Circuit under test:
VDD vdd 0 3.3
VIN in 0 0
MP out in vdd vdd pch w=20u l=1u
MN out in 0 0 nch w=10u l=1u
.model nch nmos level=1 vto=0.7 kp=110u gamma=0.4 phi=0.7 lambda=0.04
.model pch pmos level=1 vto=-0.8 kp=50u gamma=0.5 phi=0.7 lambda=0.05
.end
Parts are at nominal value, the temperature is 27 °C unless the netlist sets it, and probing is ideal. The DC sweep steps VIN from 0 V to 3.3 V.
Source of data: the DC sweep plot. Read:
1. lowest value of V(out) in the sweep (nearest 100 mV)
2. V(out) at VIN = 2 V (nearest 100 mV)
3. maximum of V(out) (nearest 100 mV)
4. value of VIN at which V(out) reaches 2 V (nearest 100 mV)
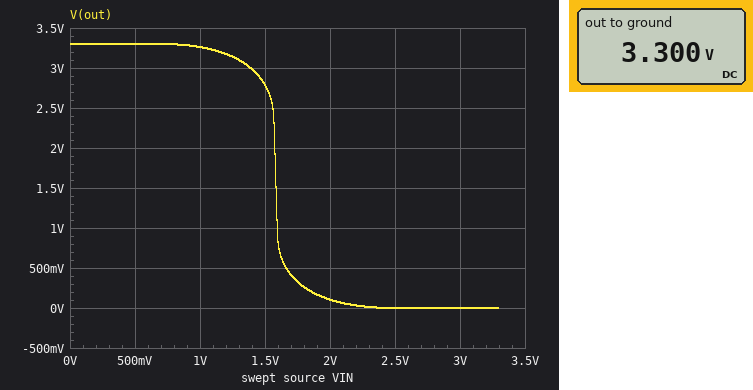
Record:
0 V
100 mV
3.3 V
1.6 V
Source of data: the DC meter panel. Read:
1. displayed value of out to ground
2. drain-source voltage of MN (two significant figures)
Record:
3.300 V
3.3 V
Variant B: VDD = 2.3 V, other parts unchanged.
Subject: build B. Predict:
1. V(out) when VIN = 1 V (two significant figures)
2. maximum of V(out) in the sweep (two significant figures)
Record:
2.2 V
2.3 V
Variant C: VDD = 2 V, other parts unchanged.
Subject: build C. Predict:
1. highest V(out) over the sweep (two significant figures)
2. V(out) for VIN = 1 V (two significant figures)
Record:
2.0 V
76 mV
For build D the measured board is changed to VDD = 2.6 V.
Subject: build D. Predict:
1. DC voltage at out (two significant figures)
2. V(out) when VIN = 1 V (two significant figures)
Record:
2.6 V
2.5 V
